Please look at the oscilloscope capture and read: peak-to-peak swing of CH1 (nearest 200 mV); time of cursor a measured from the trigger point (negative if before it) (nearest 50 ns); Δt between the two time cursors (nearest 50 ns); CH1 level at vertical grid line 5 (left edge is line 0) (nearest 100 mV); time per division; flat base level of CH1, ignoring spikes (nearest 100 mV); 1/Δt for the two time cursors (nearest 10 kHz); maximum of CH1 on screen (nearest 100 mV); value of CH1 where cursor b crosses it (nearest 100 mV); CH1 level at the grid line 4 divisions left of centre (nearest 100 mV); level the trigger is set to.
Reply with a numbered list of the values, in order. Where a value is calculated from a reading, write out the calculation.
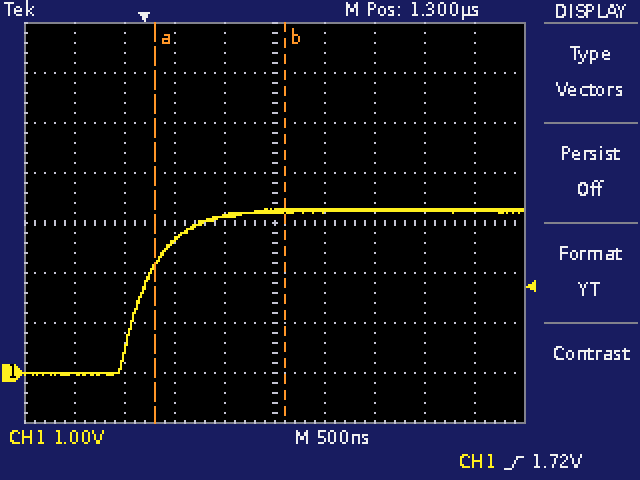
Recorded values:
1. 3.4 V
2. +100 ns
3. 1.30 µs
4. 3.2 V
5. 500 ns
6. 0.0 V
7. 1 / 1.30 µs ≈ 770 kHz
8. 3.3 V
9. 3.2 V
10. 0.0 V
11. 1.72 V
